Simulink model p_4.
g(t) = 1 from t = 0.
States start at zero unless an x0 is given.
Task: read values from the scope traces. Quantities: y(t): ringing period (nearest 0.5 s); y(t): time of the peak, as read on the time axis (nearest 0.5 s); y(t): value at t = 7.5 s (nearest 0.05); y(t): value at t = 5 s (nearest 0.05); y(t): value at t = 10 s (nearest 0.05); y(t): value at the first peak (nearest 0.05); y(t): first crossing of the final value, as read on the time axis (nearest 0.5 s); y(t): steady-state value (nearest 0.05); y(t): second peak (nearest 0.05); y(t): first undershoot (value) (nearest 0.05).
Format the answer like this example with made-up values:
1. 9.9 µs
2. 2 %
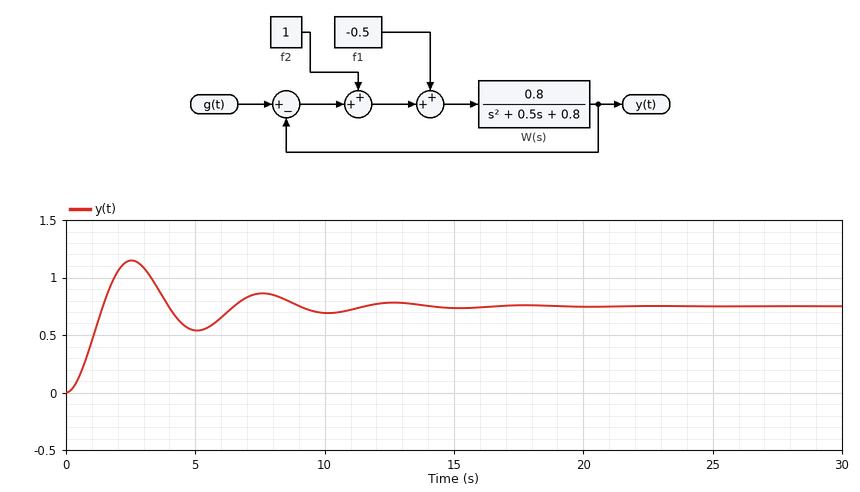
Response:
1. 5.0 s
2. 2.5 s
3. 0.85
4. 0.55
5. 0.70
6. 1.15
7. 1.5 s
8. 0.75
9. 0.85
10. 0.55
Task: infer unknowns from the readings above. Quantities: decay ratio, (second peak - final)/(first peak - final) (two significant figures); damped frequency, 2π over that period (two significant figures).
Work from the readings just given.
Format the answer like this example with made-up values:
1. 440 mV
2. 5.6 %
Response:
1. 0.25
2. 1.3 rad/s
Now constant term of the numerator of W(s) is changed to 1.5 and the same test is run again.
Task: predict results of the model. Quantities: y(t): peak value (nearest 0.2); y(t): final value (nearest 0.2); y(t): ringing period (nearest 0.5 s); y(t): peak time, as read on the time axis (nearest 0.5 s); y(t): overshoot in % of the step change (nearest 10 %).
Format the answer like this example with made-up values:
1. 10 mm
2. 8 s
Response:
1. 1.6
2. 1.0
3. 4.0 s
4. 2.0 s
5. 60 %
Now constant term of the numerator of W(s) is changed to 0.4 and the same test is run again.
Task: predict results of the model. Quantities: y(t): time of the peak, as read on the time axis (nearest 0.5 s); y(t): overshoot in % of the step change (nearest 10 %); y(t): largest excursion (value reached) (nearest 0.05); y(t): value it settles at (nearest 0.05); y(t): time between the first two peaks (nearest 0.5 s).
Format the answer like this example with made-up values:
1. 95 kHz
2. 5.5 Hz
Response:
1. 3.0 s
2. 50 %
3. 0.75
4. 0.50
5. 6.0 s
